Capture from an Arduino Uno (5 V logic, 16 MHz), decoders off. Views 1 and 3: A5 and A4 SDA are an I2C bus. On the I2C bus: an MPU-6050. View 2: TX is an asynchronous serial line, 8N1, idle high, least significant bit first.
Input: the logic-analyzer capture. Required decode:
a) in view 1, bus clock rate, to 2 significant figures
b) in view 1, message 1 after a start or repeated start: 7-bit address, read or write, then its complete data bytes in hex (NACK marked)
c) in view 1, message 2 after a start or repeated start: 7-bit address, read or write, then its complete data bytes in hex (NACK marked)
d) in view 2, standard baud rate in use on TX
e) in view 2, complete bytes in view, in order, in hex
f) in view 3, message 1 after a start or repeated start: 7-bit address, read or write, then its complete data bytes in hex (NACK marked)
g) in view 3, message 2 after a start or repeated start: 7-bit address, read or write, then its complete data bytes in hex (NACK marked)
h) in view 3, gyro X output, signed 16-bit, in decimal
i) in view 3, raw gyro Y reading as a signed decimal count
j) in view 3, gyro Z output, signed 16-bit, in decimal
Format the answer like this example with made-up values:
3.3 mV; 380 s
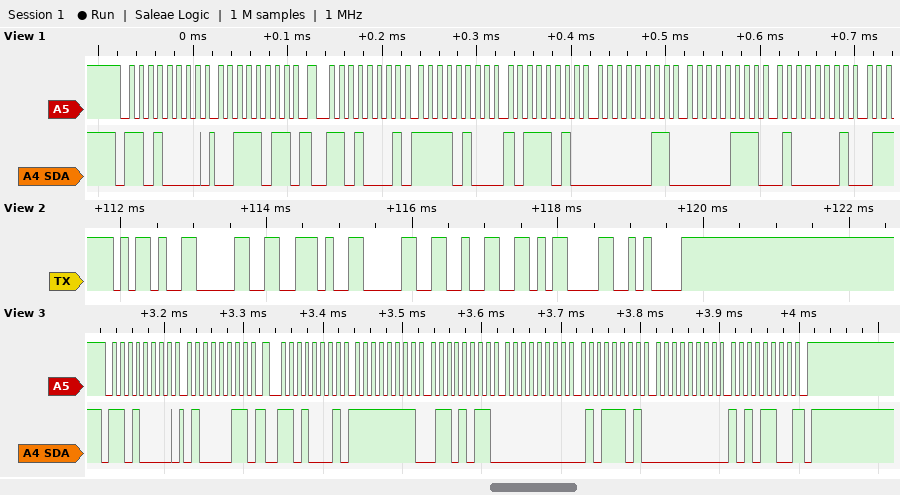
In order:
100 kHz; 0x68 write: 3B; 0x68 read: F4 BA 03 07 41; 9600 baud; 2D 30 2E 30 32 0D 0A; 0x68 write: 43; 0x68 read: FF 6B 00 5D 00 AC NACK; -149; 93; 172
